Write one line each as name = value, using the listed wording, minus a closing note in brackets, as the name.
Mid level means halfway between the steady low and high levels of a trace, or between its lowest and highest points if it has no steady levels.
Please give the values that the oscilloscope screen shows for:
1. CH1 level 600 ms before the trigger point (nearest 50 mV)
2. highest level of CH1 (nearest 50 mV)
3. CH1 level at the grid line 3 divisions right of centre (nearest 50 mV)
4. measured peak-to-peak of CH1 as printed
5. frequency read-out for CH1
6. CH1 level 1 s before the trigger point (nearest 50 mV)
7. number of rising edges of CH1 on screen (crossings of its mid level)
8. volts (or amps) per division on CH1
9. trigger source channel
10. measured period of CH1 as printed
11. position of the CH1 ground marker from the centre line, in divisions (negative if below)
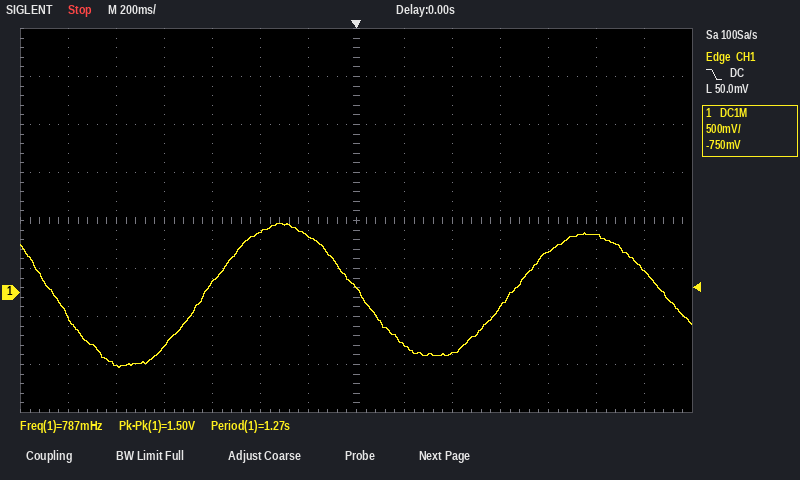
CH1 level 600 ms before the trigger point = 100 mV
highest level of CH1 = 700 mV
CH1 level at the grid line 3 divisions right of centre = -150 mV
measured peak-to-peak of CH1 as printed = 1.50 V
frequency read-out for CH1 = 787 mHz
CH1 level 1 s before the trigger point = -750 mV
number of rising edges of CH1 on screen = 2
volts (or amps) per division on CH1 = 500 mV
trigger source channel = CH1
measured period of CH1 as printed = 1.27 s
position of the CH1 ground marker from the centre line, in divisions = -1.5 div
